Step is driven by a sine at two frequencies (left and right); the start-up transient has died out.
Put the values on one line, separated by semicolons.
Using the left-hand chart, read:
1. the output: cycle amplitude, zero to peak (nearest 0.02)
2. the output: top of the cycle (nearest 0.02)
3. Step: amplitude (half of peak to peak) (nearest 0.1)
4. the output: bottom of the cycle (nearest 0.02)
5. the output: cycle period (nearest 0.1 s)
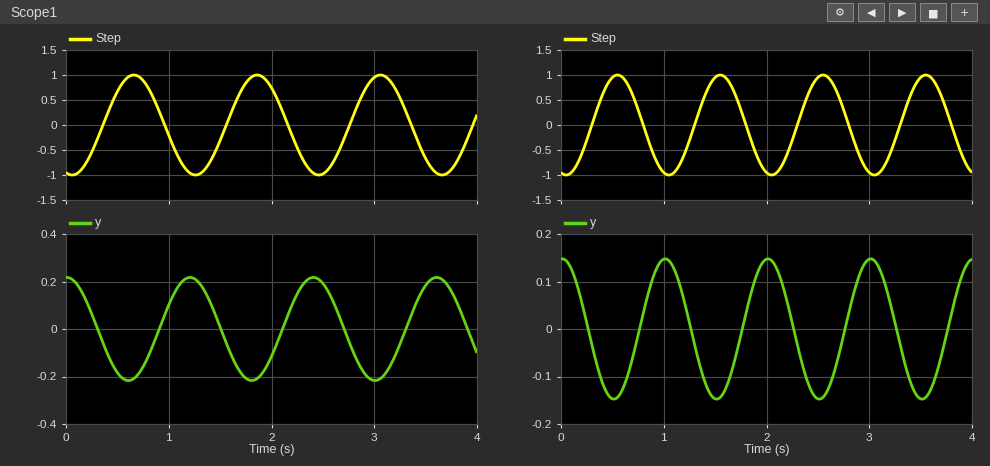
0.22; 0.22; 1.0; -0.22; 1.2 s
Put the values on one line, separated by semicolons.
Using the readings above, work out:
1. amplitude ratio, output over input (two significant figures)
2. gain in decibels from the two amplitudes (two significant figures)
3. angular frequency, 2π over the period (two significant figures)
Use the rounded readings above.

0.22; -13 dB; 5.2 rad/s
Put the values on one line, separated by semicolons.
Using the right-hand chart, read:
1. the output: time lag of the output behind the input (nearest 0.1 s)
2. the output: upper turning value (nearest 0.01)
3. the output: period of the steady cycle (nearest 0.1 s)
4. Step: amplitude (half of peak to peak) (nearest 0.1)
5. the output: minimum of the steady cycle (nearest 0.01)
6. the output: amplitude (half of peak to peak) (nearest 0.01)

0.5 s; 0.15; 1.0 s; 1.0; -0.15; 0.15
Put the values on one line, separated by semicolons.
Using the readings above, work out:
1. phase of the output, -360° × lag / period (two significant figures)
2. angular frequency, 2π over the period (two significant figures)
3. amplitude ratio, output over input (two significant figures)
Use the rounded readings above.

-180°; 6.3 rad/s; 0.15
